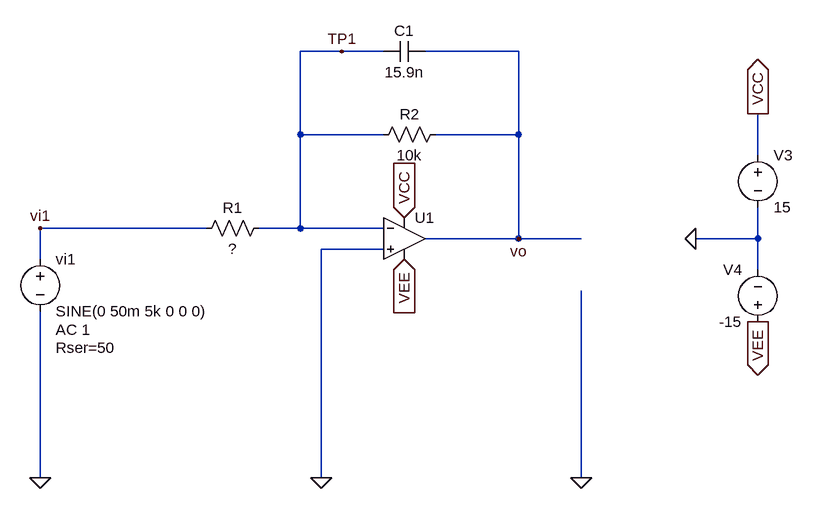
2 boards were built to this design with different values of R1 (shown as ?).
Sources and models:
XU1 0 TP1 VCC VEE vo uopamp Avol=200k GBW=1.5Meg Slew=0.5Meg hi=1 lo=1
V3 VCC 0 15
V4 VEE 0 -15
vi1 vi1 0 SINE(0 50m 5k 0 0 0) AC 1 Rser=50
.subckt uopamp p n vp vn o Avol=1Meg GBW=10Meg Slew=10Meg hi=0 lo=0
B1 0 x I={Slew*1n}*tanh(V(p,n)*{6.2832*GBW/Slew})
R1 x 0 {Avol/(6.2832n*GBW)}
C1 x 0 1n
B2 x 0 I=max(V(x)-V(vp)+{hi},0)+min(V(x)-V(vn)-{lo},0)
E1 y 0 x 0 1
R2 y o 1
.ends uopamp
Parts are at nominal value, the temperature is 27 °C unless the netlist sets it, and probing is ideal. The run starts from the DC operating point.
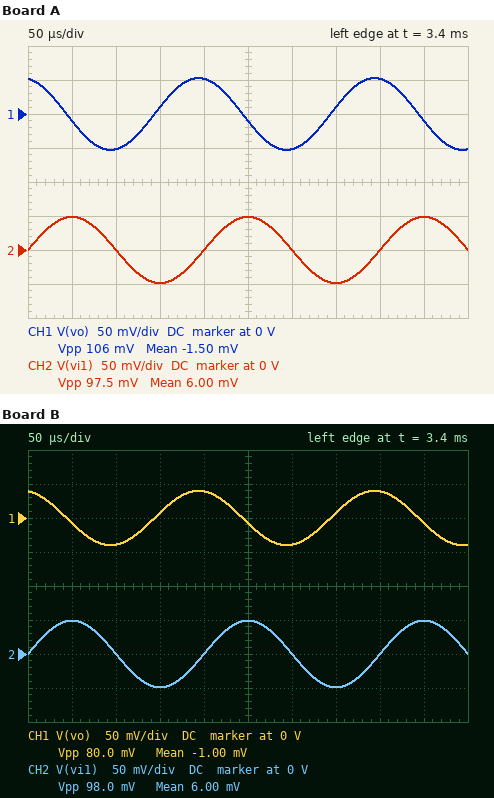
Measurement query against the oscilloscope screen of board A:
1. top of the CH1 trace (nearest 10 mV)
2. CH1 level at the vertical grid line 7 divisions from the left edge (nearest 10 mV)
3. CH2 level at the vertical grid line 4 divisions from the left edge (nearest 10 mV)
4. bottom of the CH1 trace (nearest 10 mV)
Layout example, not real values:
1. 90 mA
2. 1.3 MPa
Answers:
1. 50 mV
2. 10 mV
3. 0 V
4. -50 mV
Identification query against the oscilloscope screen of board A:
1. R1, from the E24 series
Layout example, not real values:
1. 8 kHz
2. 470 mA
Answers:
1. 1.8 kΩ
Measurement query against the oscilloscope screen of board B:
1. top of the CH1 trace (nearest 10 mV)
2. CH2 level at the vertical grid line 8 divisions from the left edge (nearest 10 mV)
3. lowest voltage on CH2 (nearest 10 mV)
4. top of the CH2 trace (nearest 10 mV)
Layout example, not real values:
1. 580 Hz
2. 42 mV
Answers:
1. 40 mV
2. 0 V
3. -50 mV
4. 50 mV
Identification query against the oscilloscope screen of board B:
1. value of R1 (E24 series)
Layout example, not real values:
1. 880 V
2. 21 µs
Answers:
1. 2.4 kΩ
